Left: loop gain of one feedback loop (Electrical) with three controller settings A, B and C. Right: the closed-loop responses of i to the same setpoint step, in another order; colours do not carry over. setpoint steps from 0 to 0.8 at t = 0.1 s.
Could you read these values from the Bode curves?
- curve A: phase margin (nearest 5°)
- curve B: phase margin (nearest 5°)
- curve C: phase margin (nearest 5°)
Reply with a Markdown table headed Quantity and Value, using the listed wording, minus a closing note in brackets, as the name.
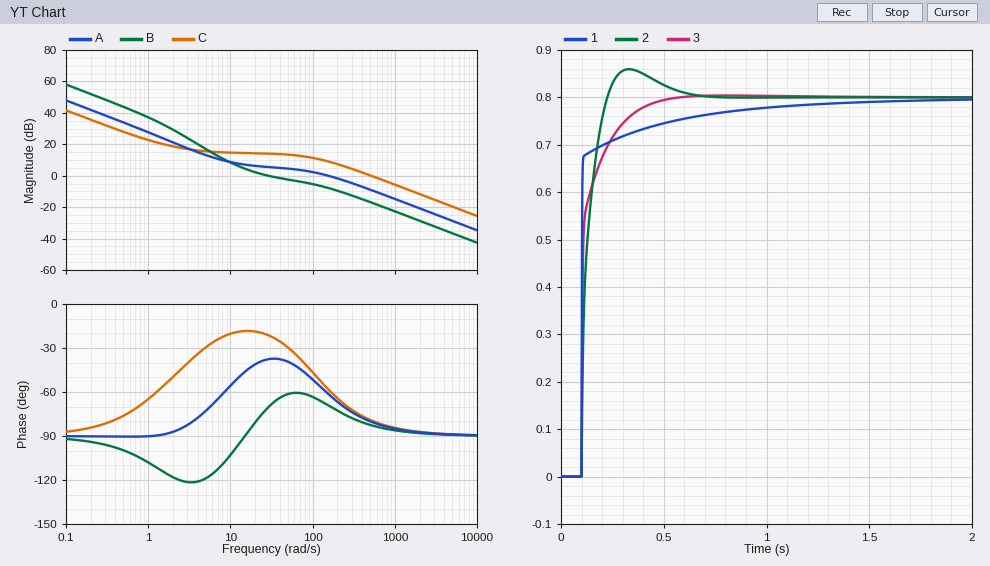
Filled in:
| Quantity | Value |
|---|---|
| curve A: phase margin | 120° |
| curve B: phase margin | 110° |
| curve C: phase margin | 100° |
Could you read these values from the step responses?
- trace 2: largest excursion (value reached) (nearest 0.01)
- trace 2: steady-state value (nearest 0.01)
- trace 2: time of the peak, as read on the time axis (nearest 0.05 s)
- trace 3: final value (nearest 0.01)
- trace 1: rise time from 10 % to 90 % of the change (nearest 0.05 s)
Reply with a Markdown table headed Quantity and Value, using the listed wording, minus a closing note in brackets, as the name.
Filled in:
| Quantity | Value |
|---|---|
| trace 2: largest excursion (value reached) | 0.86 |
| trace 2: steady-state value | 0.80 |
| trace 2: time of the peak, as read on the time axis | 0.35 s |
| trace 3: final value | 0.80 |
| trace 1: rise time from 10 % to 90 % of the change | 0.20 s |
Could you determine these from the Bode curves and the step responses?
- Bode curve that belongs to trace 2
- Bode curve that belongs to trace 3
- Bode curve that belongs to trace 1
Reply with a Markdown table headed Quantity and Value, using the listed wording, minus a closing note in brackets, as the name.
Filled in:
| Quantity | Value |
|---|---|
| Bode curve that belongs to trace 2 | B |
| Bode curve that belongs to trace 3 | A |
| Bode curve that belongs to trace 1 | C |
